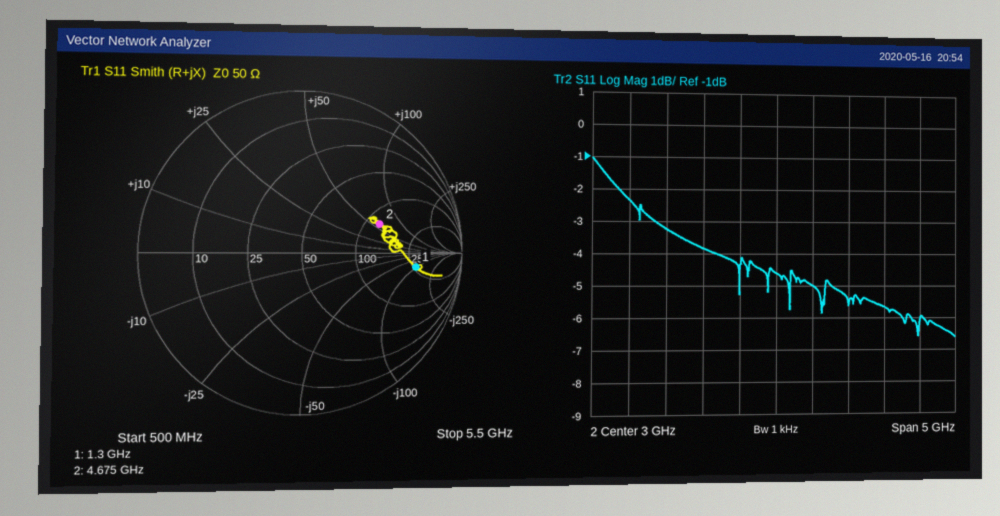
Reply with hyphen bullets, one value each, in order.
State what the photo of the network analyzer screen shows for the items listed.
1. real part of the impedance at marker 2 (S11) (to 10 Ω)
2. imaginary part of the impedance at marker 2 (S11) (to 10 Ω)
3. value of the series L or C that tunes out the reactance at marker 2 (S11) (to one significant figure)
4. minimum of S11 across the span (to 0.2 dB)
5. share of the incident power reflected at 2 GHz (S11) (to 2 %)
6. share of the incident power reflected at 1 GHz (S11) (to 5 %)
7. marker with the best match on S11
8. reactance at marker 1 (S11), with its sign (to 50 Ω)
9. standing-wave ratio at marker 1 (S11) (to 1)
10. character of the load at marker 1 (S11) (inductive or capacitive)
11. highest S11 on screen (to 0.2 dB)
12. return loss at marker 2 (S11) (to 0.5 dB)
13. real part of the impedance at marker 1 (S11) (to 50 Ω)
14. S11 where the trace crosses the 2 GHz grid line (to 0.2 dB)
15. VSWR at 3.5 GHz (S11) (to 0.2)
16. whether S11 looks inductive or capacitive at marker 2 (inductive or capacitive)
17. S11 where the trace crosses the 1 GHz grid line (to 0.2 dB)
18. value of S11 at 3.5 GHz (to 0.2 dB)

- 120 Ω
- +60 Ω
- 600 fF
- -6.6 dB
- 42 %
- 60 %
- marker 2
- -100 Ω
- 6
- capacitive
- -1.0 dB
- 6.0 dB
- 250 Ω
- -3.8 dB
- 3.6
- inductive
- -2.4 dB
- -5.0 dB
